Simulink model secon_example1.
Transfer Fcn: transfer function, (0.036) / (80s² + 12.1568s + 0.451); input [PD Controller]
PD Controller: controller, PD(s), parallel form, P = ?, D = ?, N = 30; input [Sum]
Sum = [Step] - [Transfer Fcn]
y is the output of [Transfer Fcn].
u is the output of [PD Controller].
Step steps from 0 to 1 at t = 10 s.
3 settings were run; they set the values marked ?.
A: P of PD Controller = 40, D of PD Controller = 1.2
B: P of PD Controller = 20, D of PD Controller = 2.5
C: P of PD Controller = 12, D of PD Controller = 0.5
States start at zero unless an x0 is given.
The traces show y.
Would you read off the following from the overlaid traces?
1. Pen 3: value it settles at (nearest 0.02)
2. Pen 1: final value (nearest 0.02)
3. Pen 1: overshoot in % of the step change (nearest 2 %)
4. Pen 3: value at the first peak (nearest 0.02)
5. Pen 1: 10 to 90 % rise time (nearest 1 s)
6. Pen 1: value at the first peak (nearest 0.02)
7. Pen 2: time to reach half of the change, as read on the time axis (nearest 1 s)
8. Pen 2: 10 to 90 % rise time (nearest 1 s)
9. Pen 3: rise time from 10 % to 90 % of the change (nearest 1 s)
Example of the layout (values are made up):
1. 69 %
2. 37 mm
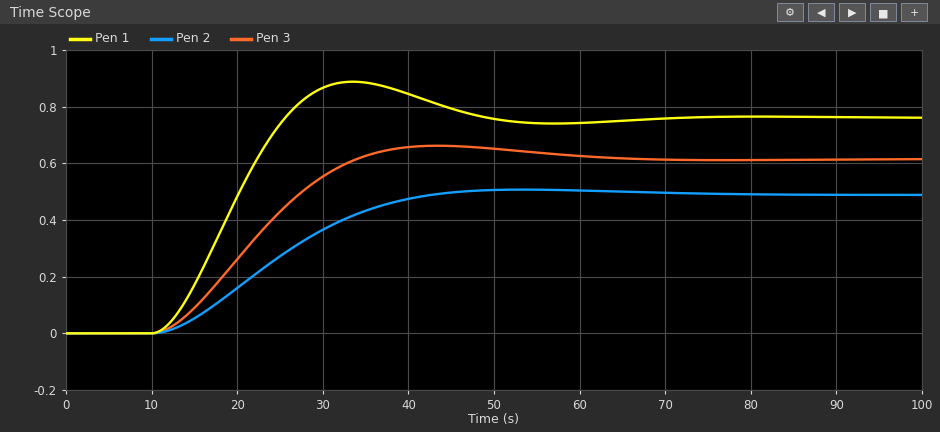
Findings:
1. 0.62
2. 0.76
3. 16 %
4. 0.66
5. 11 s
6. 0.88
7. 24 s
8. 21 s
9. 16 s
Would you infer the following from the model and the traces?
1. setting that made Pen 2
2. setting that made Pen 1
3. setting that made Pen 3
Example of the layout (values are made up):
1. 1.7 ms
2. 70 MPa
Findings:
1. C
2. A
3. B
